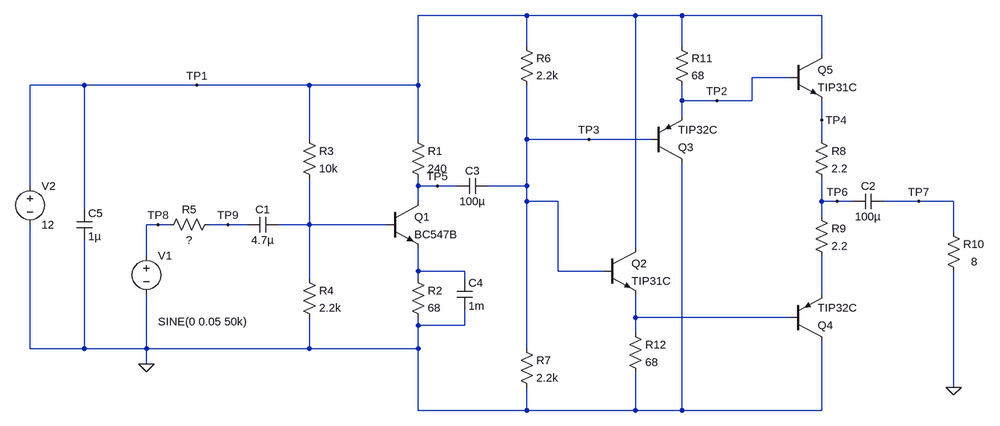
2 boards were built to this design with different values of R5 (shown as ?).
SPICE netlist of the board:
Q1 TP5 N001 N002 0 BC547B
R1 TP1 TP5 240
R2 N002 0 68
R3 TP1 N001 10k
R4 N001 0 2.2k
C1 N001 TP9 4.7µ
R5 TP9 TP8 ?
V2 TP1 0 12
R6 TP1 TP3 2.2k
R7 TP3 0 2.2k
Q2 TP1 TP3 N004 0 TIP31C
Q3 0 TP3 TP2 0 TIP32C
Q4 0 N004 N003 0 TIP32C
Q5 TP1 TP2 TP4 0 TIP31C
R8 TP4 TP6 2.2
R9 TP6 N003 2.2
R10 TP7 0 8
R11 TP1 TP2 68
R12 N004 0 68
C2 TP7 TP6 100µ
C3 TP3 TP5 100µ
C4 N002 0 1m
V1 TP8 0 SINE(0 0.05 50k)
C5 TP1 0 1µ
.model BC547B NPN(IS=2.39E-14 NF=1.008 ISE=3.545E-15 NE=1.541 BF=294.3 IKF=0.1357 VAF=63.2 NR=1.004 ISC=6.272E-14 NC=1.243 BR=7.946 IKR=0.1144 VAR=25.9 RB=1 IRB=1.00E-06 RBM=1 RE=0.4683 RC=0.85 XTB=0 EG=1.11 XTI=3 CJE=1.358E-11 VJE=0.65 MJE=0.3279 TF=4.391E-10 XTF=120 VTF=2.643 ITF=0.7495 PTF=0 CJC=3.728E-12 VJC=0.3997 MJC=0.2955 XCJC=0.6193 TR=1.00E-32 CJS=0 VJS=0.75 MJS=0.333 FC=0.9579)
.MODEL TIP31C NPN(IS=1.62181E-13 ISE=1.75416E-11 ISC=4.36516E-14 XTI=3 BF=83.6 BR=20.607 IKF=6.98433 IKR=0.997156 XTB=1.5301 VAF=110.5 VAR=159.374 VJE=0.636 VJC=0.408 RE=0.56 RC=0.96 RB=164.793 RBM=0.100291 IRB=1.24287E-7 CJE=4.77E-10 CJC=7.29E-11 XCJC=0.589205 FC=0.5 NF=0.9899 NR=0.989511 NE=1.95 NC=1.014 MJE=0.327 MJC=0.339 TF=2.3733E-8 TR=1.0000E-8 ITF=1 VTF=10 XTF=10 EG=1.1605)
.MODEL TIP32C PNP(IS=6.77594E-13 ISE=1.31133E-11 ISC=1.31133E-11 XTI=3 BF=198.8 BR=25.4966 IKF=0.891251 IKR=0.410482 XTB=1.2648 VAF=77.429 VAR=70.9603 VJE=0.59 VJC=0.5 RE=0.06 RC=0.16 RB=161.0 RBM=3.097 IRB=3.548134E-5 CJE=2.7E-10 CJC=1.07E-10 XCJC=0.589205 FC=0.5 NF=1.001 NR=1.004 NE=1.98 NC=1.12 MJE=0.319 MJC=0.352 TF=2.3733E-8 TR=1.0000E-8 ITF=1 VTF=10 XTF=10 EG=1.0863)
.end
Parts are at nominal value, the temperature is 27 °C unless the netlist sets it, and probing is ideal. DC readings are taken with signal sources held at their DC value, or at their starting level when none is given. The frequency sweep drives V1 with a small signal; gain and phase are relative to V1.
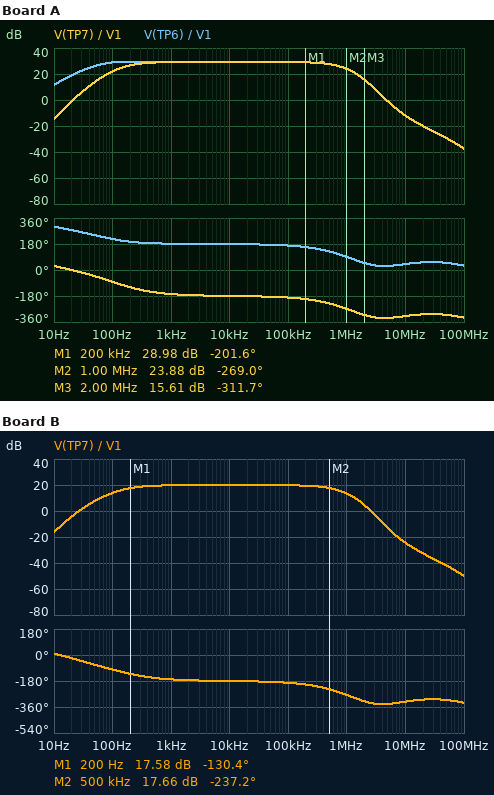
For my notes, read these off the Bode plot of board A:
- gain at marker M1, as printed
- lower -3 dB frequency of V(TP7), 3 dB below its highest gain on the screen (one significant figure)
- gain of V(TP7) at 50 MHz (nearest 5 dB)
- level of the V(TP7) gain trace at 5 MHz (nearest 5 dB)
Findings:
28.98 dB
200 Hz
-30 dB
0 dB
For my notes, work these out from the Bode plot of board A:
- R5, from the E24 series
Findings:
560 Ω
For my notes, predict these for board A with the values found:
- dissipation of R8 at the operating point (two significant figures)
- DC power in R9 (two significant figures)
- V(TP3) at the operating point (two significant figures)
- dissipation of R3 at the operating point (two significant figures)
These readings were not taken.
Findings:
1.2 mW
1.2 mW
5.6 V
9.9 mW
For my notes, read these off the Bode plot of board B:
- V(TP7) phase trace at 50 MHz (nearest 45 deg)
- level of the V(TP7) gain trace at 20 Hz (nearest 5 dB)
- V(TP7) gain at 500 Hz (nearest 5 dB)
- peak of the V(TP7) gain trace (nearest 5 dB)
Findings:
-315 deg
-5 dB
20 dB
20 dB
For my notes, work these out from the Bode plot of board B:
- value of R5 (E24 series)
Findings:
2.4 kΩ
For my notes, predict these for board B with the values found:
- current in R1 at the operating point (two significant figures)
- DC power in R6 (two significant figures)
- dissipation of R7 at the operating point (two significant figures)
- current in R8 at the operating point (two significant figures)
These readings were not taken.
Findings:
19 mA
19 mW
14 mW
23 mA
